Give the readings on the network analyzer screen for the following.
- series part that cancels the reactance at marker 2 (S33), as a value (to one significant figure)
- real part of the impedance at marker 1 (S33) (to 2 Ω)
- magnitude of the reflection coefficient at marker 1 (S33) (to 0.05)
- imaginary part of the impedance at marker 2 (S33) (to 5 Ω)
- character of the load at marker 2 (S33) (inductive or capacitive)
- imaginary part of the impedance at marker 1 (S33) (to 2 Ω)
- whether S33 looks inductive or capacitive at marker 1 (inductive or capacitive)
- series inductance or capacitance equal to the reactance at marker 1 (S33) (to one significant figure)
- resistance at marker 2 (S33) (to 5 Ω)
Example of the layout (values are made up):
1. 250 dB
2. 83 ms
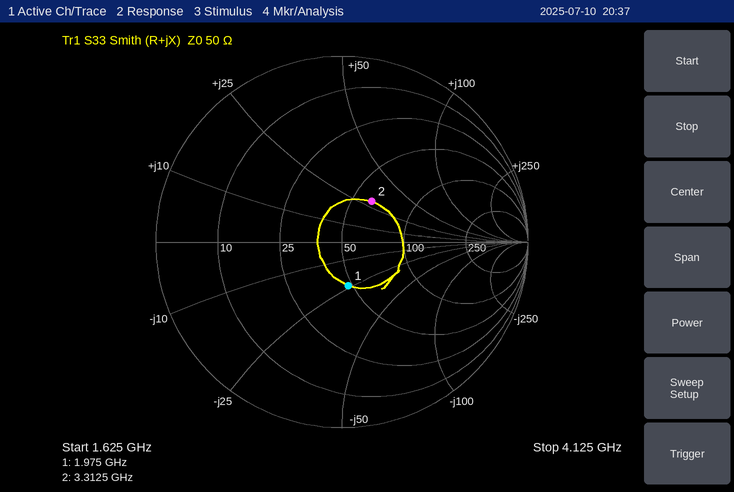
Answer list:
1. 2 pF
2. 48 Ω
3. 0.25
4. +30 Ω
5. inductive
6. -24 Ω
7. capacitive
8. 3 pF
9. 60 Ω
